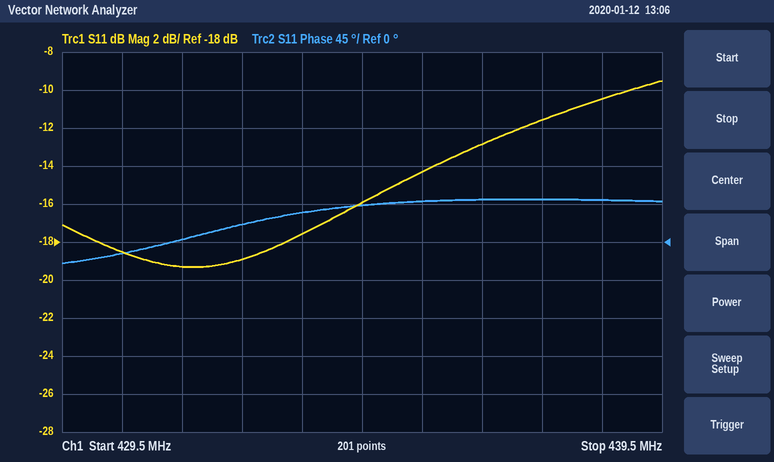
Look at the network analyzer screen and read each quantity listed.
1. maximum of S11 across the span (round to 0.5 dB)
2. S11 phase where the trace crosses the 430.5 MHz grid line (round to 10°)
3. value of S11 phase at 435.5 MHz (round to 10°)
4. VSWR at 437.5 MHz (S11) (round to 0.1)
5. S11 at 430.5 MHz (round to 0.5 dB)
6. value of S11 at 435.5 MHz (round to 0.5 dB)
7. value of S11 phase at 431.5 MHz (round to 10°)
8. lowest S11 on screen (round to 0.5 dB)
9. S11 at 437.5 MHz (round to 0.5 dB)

-9.5 dB
-10°
50°
1.7
-18.5 dB
-14.5 dB
0°
-19.5 dB
-11.5 dB
